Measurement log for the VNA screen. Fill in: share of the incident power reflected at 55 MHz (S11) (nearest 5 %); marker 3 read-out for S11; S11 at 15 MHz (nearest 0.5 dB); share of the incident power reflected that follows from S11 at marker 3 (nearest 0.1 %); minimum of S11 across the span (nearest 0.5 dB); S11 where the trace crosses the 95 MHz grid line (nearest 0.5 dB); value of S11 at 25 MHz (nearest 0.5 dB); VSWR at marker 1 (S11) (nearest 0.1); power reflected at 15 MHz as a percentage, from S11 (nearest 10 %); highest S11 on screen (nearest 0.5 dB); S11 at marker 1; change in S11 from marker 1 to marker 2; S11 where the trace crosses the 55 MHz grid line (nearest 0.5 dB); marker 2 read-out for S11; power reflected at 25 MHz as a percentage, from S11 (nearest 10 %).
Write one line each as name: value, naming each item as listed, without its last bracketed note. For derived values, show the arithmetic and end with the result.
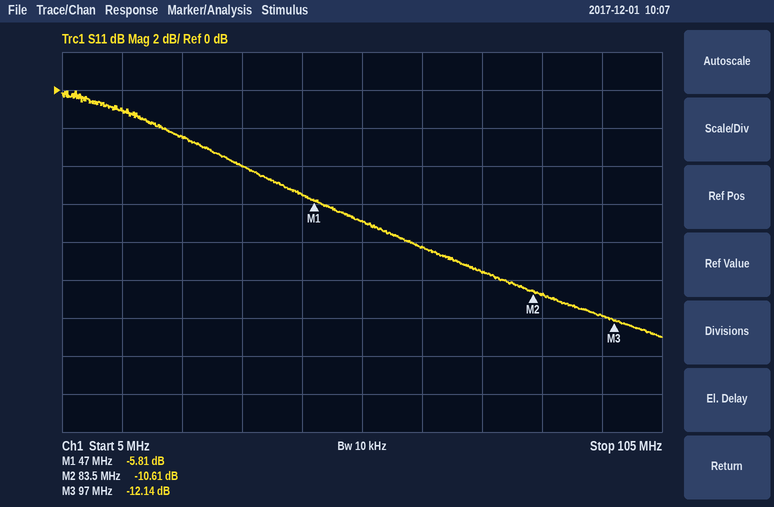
share of the incident power reflected at 55 MHz (S11): 10^(-7/10) ≈ 20 %
marker 3 read-out for S11: -12.14 dB
S11 at 15 MHz: -1.0 dB
share of the incident power reflected that follows from S11 at marker 3: 10^(-12.14/10) ≈ 6.1 %
minimum of S11 across the span: -13.0 dB
S11 where the trace crosses the 95 MHz grid line: -12.0 dB
value of S11 at 25 MHz: -2.5 dB
VSWR at marker 1 (S11): (1 + 0.5123)/(1 − 0.5123) ≈ 3.1
power reflected at 15 MHz as a percentage, from S11: 10^(-1/10) ≈ 79.4 %, so 80 % to the nearest 10 %
highest S11 on screen: 0.0 dB
S11 at marker 1: -5.81 dB
change in S11 from marker 1 to marker 2: -10.61 − (-5.81) = -4.80 dB
S11 where the trace crosses the 55 MHz grid line: -7.0 dB
marker 2 read-out for S11: -10.61 dB
power reflected at 25 MHz as a percentage, from S11: 10^(-2.5/10) ≈ 56.2 %, so 60 % to the nearest 10 %
